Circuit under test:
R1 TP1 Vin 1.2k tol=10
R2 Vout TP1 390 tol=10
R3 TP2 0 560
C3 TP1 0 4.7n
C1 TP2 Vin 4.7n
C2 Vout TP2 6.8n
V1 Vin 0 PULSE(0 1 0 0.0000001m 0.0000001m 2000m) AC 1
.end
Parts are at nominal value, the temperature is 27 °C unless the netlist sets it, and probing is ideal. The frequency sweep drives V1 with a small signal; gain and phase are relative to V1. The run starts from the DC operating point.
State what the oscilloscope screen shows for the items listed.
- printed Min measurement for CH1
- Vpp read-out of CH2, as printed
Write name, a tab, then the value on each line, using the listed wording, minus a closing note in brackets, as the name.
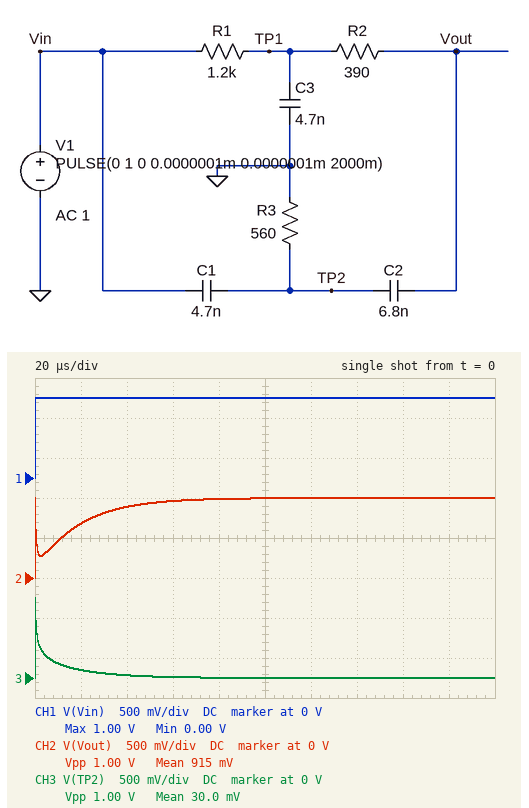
printed Min measurement for CH1	0.00 V
Vpp read-out of CH2, as printed	1.00 V
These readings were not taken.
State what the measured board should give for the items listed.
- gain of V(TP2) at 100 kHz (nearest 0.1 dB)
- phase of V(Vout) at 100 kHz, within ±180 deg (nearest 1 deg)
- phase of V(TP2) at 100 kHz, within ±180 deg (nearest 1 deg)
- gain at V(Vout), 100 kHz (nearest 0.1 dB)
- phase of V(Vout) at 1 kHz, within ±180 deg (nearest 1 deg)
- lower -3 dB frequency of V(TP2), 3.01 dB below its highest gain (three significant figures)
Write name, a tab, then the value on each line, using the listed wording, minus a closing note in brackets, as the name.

gain of V(TP2) at 100 kHz	-4.7 dB
phase of V(Vout) at 100 kHz, within ±180 deg	38 deg
phase of V(TP2) at 100 kHz, within ±180 deg	27 deg
gain at V(Vout), 100 kHz	-8.4 dB
phase of V(Vout) at 1 kHz, within ±180 deg	-6 deg
lower -3 dB frequency of V(TP2), 3.01 dB below its highest gain	182 kHz
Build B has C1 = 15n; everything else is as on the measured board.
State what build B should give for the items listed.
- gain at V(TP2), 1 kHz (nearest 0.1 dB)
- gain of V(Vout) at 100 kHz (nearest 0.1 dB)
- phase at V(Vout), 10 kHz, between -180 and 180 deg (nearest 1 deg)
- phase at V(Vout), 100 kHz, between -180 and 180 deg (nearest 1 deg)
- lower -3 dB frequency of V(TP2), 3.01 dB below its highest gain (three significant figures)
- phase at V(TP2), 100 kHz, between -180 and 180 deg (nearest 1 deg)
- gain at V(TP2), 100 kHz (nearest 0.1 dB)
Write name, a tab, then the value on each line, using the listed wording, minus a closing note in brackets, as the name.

gain at V(TP2), 1 kHz	-22.4 dB
gain of V(Vout) at 100 kHz	-4.3 dB
phase at V(Vout), 10 kHz, between -180 and 180 deg	-31 deg
phase at V(Vout), 100 kHz, between -180 and 180 deg	23 deg
lower -3 dB frequency of V(TP2), 3.01 dB below its highest gain	24.5 kHz
phase at V(TP2), 100 kHz, between -180 and 180 deg	12 deg
gain at V(TP2), 100 kHz	-1.3 dB
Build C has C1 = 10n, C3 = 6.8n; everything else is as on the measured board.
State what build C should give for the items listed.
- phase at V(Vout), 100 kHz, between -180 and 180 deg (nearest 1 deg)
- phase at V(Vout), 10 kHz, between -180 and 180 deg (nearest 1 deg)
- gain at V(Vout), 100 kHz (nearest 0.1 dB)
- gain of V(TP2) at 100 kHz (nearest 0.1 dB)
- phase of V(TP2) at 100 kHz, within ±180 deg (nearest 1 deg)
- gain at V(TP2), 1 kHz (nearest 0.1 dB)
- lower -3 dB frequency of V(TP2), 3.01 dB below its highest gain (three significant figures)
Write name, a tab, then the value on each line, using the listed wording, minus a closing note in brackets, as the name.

phase at V(Vout), 100 kHz, between -180 and 180 deg	35 deg
phase at V(Vout), 10 kHz, between -180 and 180 deg	-42 deg
gain at V(Vout), 100 kHz	-5.5 dB
gain of V(TP2) at 100 kHz	-2.3 dB
phase of V(TP2) at 100 kHz, within ±180 deg	19 deg
gain at V(TP2), 1 kHz	-24.6 dB
lower -3 dB frequency of V(TP2), 3.01 dB below its highest gain	63.7 kHz
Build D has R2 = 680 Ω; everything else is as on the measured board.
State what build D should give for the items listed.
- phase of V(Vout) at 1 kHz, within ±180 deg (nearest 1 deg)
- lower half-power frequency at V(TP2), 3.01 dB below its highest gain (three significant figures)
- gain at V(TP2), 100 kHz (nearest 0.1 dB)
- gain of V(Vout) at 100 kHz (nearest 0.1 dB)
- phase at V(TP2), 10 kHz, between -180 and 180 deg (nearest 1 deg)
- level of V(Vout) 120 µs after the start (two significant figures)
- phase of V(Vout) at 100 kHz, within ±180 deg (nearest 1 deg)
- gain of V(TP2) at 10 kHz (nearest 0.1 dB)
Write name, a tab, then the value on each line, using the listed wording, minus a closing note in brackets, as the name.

phase of V(Vout) at 1 kHz, within ±180 deg	-7 deg
lower half-power frequency at V(TP2), 3.01 dB below its highest gain	134 kHz
gain at V(TP2), 100 kHz	-4.1 dB
gain of V(Vout) at 100 kHz	-6.3 dB
phase at V(TP2), 10 kHz, between -180 and 180 deg	48 deg
level of V(Vout) 120 µs after the start	1.0 V
phase of V(Vout) at 100 kHz, within ±180 deg	44 deg
gain of V(TP2) at 10 kHz	-11.7 dB
